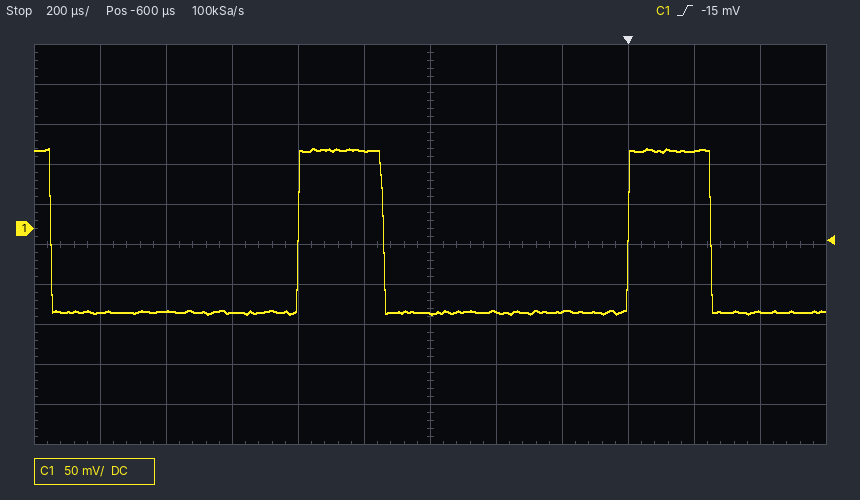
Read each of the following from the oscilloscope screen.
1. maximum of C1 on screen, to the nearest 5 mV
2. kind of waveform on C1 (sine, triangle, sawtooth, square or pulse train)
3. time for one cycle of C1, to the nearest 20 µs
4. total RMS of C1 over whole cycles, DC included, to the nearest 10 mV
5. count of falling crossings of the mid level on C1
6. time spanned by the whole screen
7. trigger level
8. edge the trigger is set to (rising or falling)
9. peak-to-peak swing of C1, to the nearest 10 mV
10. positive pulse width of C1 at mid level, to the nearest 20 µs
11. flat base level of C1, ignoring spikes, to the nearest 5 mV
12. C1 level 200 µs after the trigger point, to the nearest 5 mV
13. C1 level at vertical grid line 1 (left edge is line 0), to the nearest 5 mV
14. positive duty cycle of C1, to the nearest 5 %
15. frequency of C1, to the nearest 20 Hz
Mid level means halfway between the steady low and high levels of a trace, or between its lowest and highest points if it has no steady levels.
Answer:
100 mV
pulse train
1.00 ms
100 mV
3
2.4 ms
-15 mV
rising
210 mV
260 µs
-105 mV
95 mV
-105 mV
25 %
1.00 kHz
